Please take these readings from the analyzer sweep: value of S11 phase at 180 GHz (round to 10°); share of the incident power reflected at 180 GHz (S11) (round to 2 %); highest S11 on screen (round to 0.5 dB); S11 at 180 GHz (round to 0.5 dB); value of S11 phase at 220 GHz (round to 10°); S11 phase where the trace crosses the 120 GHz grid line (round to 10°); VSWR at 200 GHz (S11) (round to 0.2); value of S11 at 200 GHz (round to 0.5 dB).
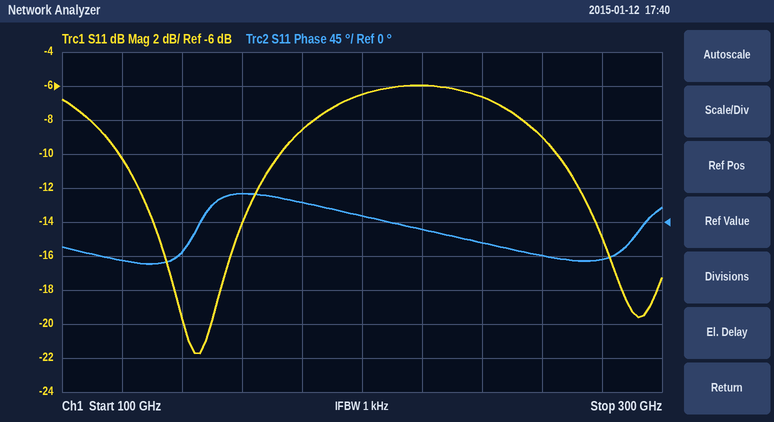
30°
14 %
-6.0 dB
-8.5 dB
-10°
-50°
2.8
-6.5 dB
